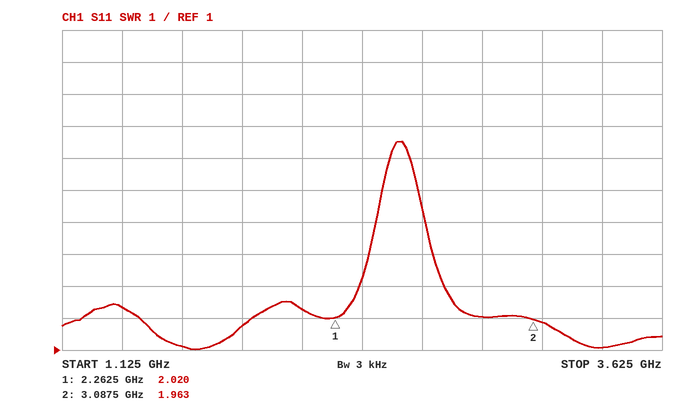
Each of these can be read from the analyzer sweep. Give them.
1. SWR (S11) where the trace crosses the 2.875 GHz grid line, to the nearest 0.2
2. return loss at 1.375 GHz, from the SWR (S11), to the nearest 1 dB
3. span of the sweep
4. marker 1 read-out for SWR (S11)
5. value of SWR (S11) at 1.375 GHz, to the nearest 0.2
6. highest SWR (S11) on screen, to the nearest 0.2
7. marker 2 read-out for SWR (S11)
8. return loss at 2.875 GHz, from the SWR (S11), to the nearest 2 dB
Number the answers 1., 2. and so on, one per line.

1. 2.0
2. 8 dB
3. 2.5 GHz
4. 2.020
5. 2.4
6. 7.6
7. 1.963
8. 10 dB
